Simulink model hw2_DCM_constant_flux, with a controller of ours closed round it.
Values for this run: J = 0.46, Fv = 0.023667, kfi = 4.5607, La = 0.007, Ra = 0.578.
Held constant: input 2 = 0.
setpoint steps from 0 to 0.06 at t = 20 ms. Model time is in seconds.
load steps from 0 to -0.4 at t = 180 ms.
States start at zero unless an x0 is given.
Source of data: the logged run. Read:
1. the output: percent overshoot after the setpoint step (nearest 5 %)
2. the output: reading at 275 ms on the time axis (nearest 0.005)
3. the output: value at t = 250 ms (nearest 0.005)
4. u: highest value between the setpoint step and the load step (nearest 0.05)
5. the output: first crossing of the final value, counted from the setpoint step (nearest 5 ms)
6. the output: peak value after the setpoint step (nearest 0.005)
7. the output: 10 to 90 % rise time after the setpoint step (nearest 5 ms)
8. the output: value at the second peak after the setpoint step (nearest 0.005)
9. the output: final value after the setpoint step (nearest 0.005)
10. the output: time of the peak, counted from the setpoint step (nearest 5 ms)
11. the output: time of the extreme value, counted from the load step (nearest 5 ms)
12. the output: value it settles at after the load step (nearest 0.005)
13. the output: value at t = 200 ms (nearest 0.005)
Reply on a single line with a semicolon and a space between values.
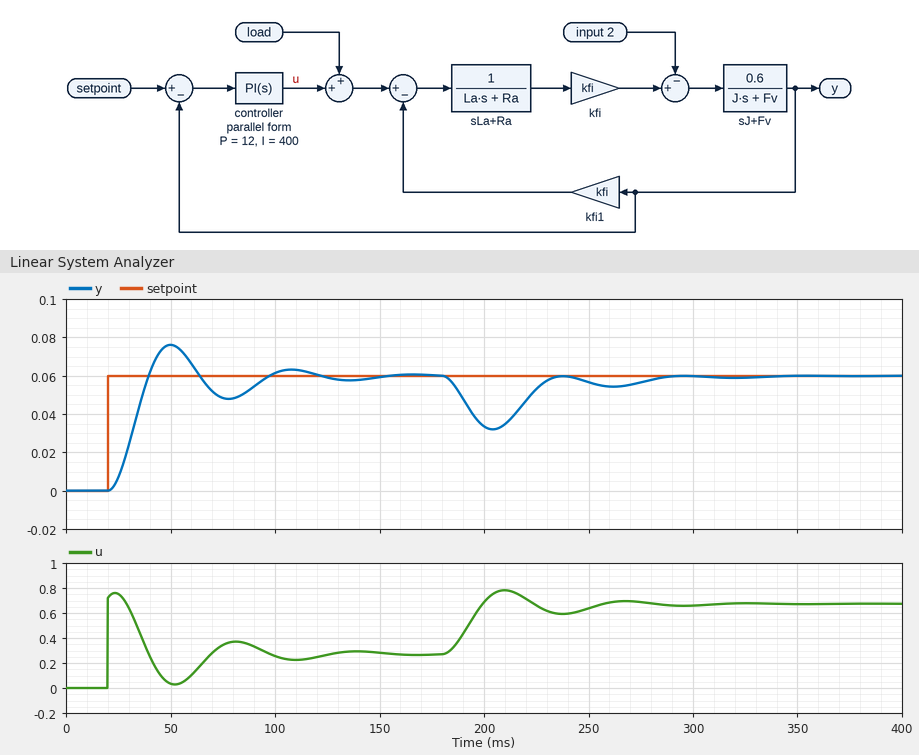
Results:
25 %; 0.055; 0.055; 0.75; 20 ms; 0.075; 15 ms; 0.065; 0.060; 30 ms; 25 ms; 0.060; 0.035
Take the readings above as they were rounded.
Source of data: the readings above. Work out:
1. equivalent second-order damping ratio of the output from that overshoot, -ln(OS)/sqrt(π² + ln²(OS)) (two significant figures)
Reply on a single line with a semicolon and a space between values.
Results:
0.40
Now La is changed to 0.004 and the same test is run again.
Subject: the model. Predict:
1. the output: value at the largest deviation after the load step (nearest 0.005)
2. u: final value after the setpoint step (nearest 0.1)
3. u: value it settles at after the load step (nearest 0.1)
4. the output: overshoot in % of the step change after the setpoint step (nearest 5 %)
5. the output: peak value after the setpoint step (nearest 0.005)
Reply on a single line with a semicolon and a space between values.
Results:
0.035; 0.3; 0.7; 10 %; 0.065
